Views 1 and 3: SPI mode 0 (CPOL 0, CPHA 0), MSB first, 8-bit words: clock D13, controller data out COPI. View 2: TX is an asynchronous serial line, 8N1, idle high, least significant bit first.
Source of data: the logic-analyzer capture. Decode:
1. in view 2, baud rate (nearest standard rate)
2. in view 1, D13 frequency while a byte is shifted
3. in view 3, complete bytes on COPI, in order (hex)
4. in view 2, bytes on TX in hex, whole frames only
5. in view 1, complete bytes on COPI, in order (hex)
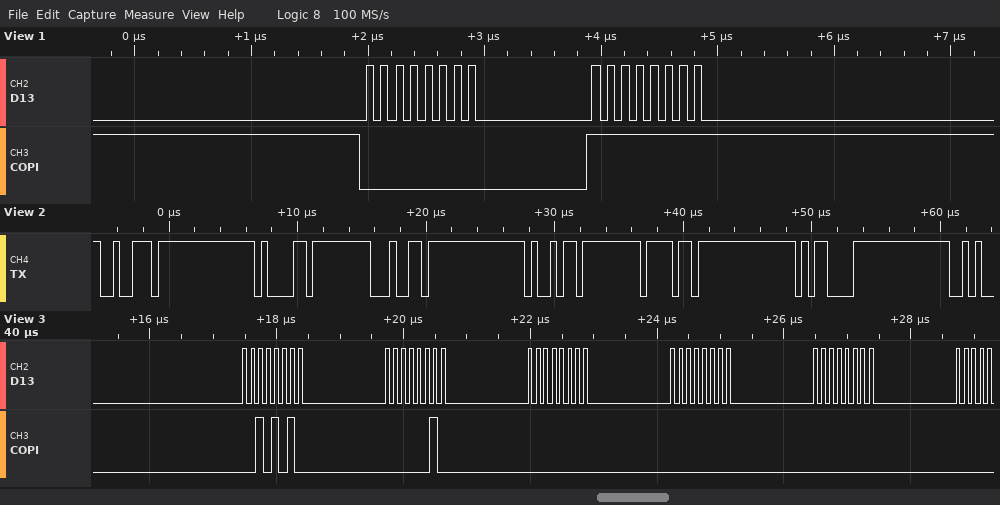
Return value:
2000000 baud
8 MHz
2A 02 00 00 00
72 61 64 69 6F 0D
0x00 0xFF
